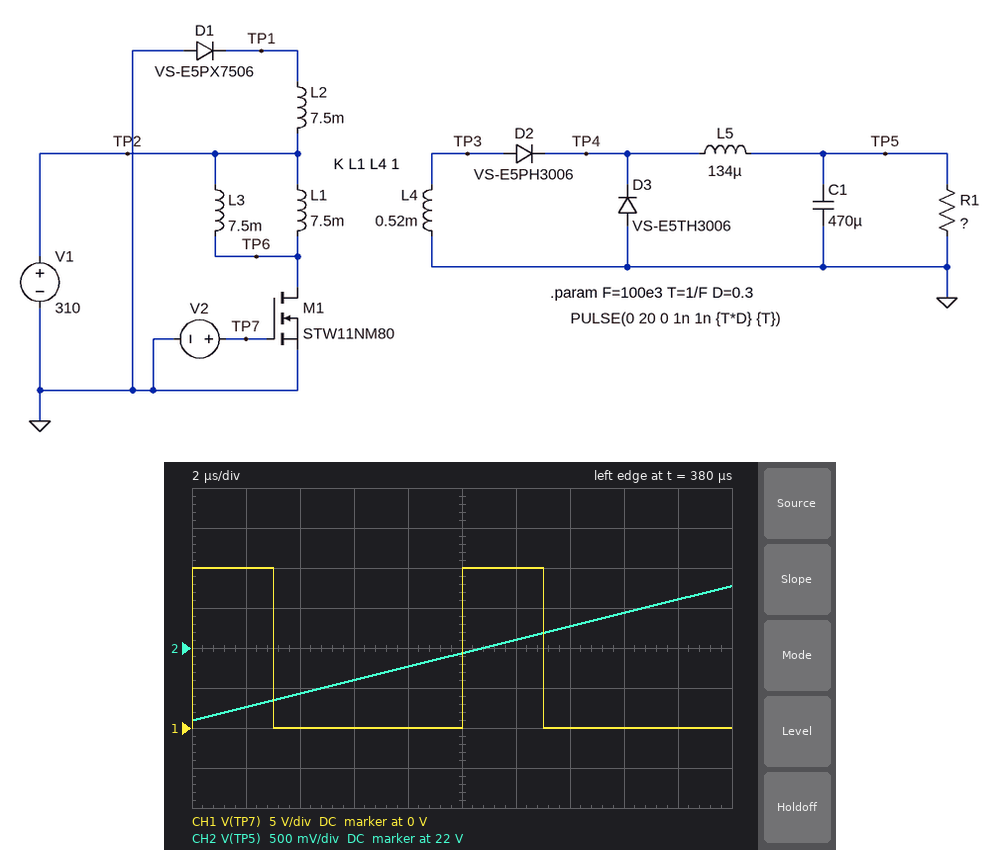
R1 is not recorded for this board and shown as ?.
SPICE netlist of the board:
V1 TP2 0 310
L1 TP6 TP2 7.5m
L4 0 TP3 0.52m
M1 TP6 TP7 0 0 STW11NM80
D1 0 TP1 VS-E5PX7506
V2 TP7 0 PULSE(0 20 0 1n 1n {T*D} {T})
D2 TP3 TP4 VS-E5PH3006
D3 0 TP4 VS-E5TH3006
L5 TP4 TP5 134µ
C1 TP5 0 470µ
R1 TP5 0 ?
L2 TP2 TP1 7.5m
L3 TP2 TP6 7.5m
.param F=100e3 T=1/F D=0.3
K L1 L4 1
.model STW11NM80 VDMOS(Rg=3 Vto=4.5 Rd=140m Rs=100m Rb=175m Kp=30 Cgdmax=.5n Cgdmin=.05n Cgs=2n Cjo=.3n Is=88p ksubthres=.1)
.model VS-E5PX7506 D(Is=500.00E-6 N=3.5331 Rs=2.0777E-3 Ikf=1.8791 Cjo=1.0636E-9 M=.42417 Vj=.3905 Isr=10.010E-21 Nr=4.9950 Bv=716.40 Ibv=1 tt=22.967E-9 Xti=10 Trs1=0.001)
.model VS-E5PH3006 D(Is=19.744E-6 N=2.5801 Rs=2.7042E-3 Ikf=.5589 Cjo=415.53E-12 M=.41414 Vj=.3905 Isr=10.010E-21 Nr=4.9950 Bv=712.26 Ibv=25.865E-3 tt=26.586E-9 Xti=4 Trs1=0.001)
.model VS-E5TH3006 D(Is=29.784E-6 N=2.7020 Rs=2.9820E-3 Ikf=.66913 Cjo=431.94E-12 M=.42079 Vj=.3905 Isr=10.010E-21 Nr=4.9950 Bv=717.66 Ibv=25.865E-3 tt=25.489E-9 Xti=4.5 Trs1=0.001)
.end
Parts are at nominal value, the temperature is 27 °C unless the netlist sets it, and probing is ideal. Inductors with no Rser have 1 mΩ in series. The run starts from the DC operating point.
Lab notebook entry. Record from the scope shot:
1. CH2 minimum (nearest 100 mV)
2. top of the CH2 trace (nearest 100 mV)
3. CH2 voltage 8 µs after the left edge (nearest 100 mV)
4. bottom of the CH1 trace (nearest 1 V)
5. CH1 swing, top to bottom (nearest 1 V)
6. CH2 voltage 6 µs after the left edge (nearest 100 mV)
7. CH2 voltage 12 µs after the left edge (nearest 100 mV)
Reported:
21.1 V
22.8 V
21.8 V
0 V
20 V
21.6 V
22.1 V
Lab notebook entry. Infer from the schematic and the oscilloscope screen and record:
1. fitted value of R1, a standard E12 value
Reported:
4.7 Ω
